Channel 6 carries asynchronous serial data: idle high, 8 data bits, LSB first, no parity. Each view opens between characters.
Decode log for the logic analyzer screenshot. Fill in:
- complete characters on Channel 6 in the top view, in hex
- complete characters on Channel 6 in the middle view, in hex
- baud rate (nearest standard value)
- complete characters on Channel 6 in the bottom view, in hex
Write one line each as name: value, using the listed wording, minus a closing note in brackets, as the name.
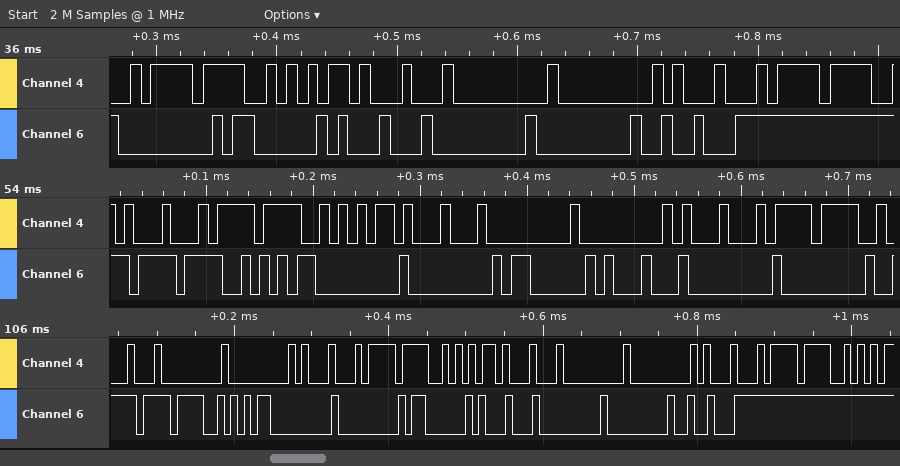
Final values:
complete characters on Channel 6 in the top view, in hex: 00, 03, 11, 00, 00, 12
complete characters on Channel 6 in the middle view, in hex: EF, AA, 00, 00, 03, 11, 00, 00
baud rate: 115200 baud
complete characters on Channel 6 in the bottom view, in hex: EF, AA, 00, 00, 03, 11, 00, 00, 12
